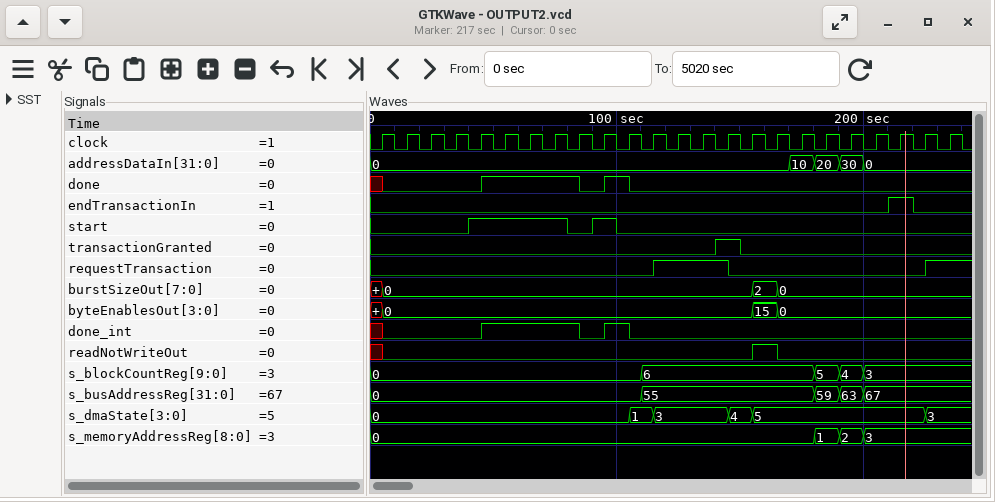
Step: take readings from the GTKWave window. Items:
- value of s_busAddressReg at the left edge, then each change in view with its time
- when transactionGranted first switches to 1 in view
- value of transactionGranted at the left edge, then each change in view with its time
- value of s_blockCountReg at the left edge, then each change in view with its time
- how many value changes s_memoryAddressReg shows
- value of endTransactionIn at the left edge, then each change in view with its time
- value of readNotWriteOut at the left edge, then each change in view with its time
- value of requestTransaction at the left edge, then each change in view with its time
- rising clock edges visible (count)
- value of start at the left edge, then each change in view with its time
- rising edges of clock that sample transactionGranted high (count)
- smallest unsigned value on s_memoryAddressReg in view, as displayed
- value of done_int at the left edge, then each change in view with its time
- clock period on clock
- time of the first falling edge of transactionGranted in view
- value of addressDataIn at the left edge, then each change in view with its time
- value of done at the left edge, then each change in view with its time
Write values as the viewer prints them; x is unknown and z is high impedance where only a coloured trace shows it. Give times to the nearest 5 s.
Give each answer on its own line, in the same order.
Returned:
0, 55 at 110 s, 59 at 180 s, 63 at 190 s, 67 at 200 s
140 s
0, 1 at 140 s, 0 at 150 s
0, 6 at 110 s, 5 at 180 s, 4 at 190 s, 3 at 200 s
3
0, 1 at 210 s, 0 at 220 s
x, 0 at 5 s, 1 at 155 s, 0 at 165 s
0, 1 at 115 s, 0 at 145 s, 1 at 225 s
24
0, 1 at 40 s, 0 at 80 s, 1 at 90 s, 0 at 100 s
1
0
x, 0 at 5 s, 1 at 45 s, 0 at 85 s, 1 at 95 s, 0 at 105 s
10 s
150 s
0, 10 at 170 s, 20 at 180 s, 30 at 190 s, 0 at 200 s
x, 0 at 5 s, 1 at 45 s, 0 at 85 s, 1 at 95 s, 0 at 105 s
